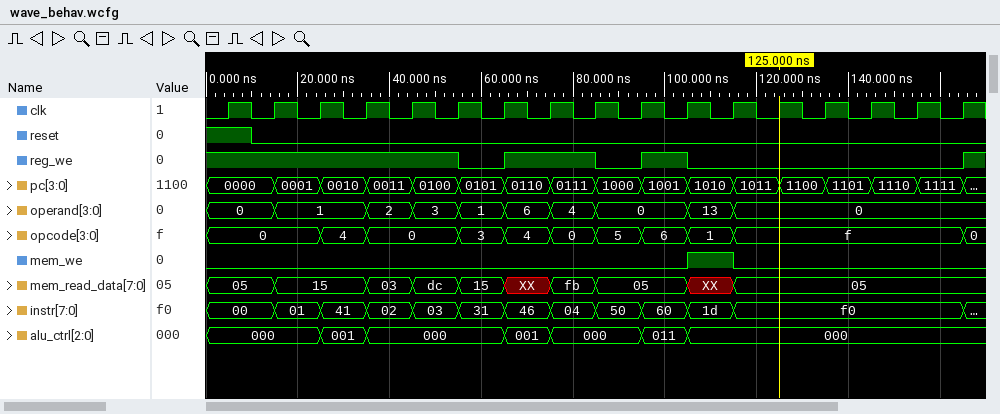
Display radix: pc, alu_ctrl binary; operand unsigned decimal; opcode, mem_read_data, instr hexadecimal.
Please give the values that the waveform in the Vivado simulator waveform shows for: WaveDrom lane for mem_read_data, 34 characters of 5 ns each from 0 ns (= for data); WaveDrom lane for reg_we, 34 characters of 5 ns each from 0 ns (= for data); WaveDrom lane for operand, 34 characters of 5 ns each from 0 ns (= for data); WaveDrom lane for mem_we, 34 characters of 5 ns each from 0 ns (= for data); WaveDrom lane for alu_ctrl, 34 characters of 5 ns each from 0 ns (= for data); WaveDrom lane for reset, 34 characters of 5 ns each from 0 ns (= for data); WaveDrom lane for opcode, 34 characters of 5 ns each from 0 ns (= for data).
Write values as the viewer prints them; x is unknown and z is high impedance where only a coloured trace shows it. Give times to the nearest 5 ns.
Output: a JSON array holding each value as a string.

["{name: 'mem_read_data', wave: '=..=...=.=.=.x.=.=...x.=..........', data: '05 15 03 dc 15 fb 05 05'}", "{name: 'reg_we', wave: '1..........0.1...0.1.0...........1'}", "{name: 'operand', wave: '=..=...=.=.=.=.=.=...=.=..........', data: '0 1 2 3 1 6 4 0 13 0'}", "{name: 'mem_we', wave: '0....................1.0..........'}", "{name: 'alu_ctrl', wave: '=....=.=.....=.=...=.=............', data: '000 001 000 001 000 011 000'}", "{name: 'reset', wave: '1.0...............................'}", "{name: 'opcode', wave: '=....=.=...=.=.=.=.=.=.=.........=', data: '0 4 0 3 4 0 5 6 1 f 0'}"]
